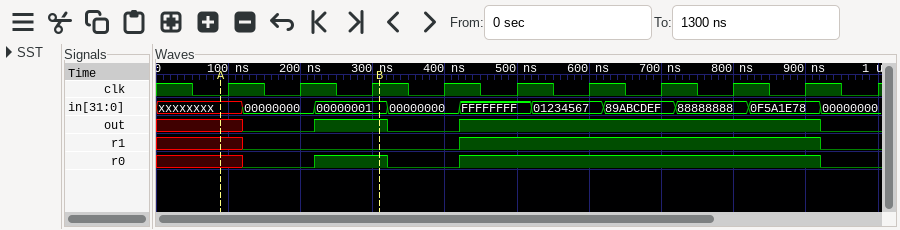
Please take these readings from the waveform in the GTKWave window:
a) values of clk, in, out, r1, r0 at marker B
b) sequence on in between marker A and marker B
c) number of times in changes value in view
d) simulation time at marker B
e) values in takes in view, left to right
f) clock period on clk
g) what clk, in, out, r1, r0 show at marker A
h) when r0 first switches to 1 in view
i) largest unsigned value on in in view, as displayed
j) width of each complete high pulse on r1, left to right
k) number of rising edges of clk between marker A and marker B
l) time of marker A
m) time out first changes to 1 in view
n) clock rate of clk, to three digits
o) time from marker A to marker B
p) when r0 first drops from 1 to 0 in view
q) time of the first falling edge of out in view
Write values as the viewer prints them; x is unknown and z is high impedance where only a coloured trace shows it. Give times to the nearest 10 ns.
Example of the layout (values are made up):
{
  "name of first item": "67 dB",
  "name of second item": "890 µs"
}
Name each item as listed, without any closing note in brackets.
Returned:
{
  "values of clk, in, out, r1, r0 at marker B": "clk=1, in=00000001, out=1, r1=0, r0=1",
  "sequence on in between marker A and marker B": "xxxxxxxx, 00000000, 00000001",
  "number of times in changes value in view": "9",
  "simulation time at marker B": "310 ns",
  "values in takes in view, left to right": "xxxxxxxx, 00000000, 00000001, 00000000, FFFFFFFF, 01234567, 89ABCDEF, 88888888, 0F5A1E78, 00000000",
  "clock period on clk": "100 ns",
  "what clk, in, out, r1, r0 show at marker A": "clk=0, in=xxxxxxxx, out=x, r1=x, r0=x",
  "when r0 first switches to 1 in view": "220 ns",
  "largest unsigned value on in in view, as displayed": "FFFFFFFF",
  "width of each complete high pulse on r1, left to right": "500 ns",
  "number of rising edges of clk between marker A and marker B": "3",
  "time of marker A": "90 ns",
  "time out first changes to 1 in view": "220 ns",
  "clock rate of clk, to three digits": "10.0 MHz",
  "time from marker A to marker B": "220 ns",
  "when r0 first drops from 1 to 0 in view": "320 ns",
  "time of the first falling edge of out in view": "320 ns"
}
